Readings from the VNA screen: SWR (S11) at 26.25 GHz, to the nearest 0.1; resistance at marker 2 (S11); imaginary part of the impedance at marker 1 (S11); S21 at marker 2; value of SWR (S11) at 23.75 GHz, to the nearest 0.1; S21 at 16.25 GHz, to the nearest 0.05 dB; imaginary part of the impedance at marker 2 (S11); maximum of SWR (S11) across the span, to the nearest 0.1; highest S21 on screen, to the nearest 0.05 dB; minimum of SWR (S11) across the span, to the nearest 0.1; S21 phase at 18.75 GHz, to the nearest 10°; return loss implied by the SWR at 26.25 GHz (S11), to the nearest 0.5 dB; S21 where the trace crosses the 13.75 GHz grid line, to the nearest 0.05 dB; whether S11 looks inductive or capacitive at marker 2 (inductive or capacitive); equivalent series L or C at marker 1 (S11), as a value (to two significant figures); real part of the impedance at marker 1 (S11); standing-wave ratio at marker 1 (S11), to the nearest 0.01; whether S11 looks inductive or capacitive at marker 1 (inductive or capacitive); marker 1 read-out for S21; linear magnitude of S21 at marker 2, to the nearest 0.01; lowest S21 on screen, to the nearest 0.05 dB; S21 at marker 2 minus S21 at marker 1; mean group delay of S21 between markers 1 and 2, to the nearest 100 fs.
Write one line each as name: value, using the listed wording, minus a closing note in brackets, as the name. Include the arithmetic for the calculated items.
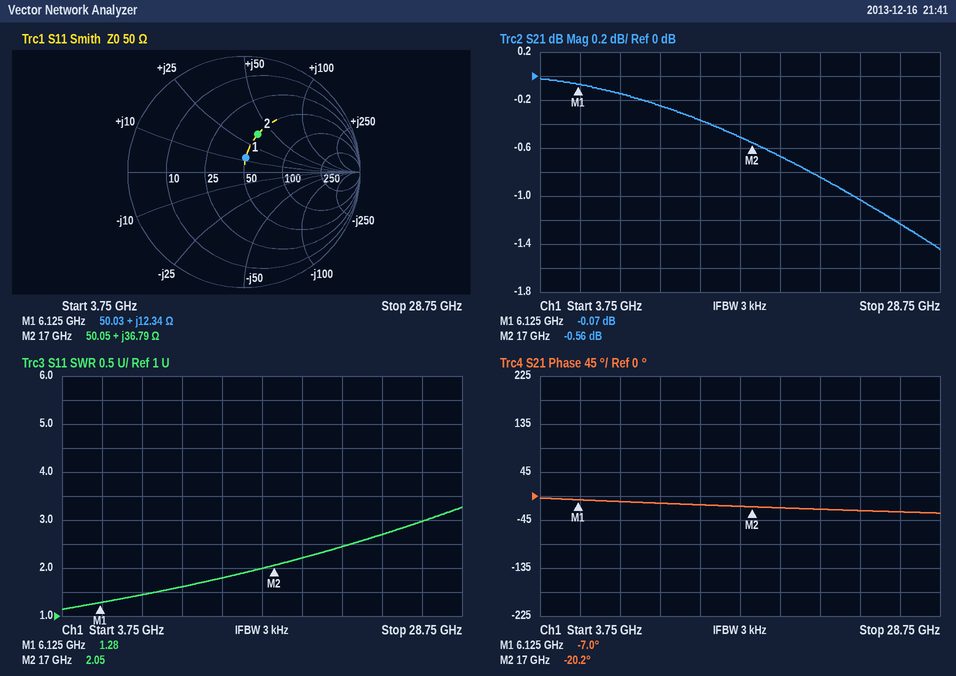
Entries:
SWR (S11) at 26.25 GHz, to the nearest 0.1: 3.0
resistance at marker 2: 50.05 Ω
imaginary part of the impedance at marker 1: +12.34 Ω
S21 at marker 2: -0.56 dB
value of SWR (S11) at 23.75 GHz, to the nearest 0.1: 2.7
S21 at 16.25 GHz, to the nearest 0.05 dB: -0.50 dB
imaginary part of the impedance at marker 2: +36.79 Ω
maximum of SWR (S11) across the span, to the nearest 0.1: 3.3
highest S21 on screen, to the nearest 0.05 dB: 0.00 dB
minimum of SWR (S11) across the span, to the nearest 0.1: 1.1
S21 phase at 18.75 GHz, to the nearest 10°: -20°
return loss implied by the SWR at 26.25 GHz (S11), to the nearest 0.5 dB: −20 log10((3 − 1)/(3 + 1)) ≈ 6.0 dB
S21 where the trace crosses the 13.75 GHz grid line, to the nearest 0.05 dB: -0.35 dB
whether S11 looks inductive or capacitive at marker 2: inductive
equivalent series L or C at marker 1 (S11), as a value: L = 12.34 Ω/(2π × 6.125 GHz) ≈ 321 pH, so 320 pH to two significant figures
real part of the impedance at marker 1: 50.03 Ω
standing-wave ratio at marker 1 (S11), to the nearest 0.01: 1.28
whether S11 looks inductive or capacitive at marker 1: inductive
marker 1 read-out for S21: -0.07 dB
linear magnitude of S21 at marker 2, to the nearest 0.01: 10^(-0.56/20) ≈ 0.94
lowest S21 on screen, to the nearest 0.05 dB: -1.45 dB
S21 at marker 2 minus S21 at marker 1: -0.56 − (-0.07) = -0.49 dB
mean group delay of S21 between markers 1 and 2, to the nearest 100 fs: −(-20.2° − (-7°))/(360° × 10.875 GHz) ≈ 3.4 ps
